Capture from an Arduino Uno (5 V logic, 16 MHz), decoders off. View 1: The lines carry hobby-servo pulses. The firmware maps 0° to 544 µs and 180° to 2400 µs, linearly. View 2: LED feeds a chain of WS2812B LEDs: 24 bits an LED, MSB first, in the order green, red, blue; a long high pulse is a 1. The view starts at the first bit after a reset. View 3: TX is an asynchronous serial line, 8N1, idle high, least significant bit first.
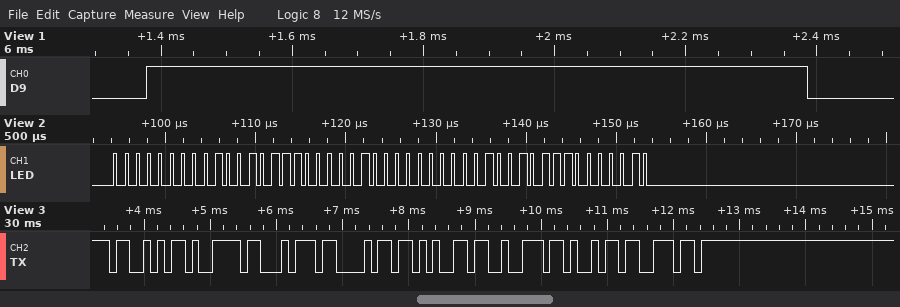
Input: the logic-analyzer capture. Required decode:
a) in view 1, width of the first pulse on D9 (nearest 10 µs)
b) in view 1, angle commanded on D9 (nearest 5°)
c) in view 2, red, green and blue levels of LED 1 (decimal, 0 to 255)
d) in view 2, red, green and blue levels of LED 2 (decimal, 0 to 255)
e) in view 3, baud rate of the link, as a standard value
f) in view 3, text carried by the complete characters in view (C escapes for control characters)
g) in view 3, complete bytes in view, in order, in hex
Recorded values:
1010 µs
45°
75, 0, 130
75, 0, 130
9600 baud
"Sytherin"
0x53 0x79 0x74 0x68 0x65 0x72 0x69 0x6E
